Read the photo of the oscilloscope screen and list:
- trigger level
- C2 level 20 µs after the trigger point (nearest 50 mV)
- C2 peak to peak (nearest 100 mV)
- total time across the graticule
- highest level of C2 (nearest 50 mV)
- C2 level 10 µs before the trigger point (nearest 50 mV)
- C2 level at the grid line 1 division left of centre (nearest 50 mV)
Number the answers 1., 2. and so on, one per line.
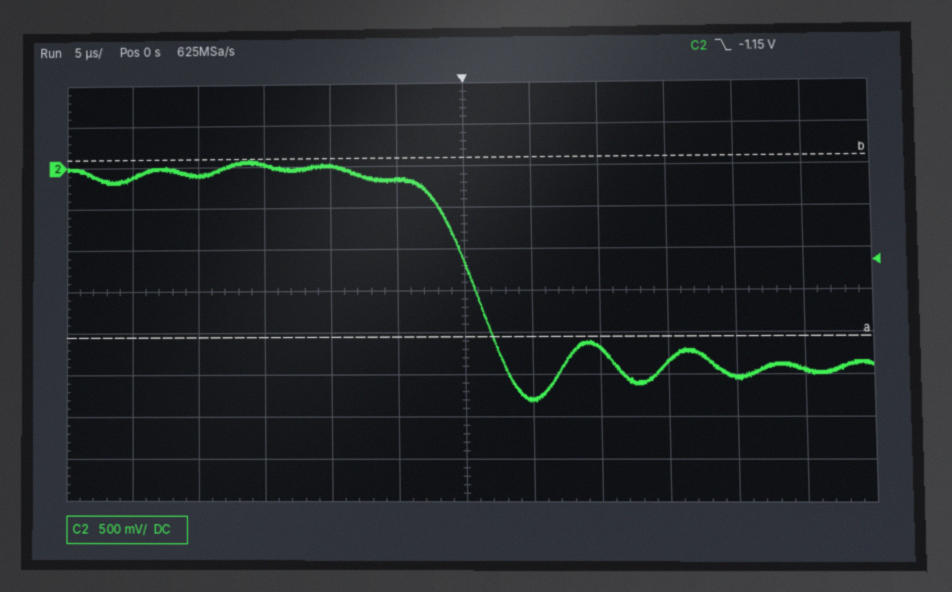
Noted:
1. -1.15 V
2. -2.55 V
3. 2.90 V
4. 60 µs
5. 100 mV
6. 0 mV
7. -150 mV
